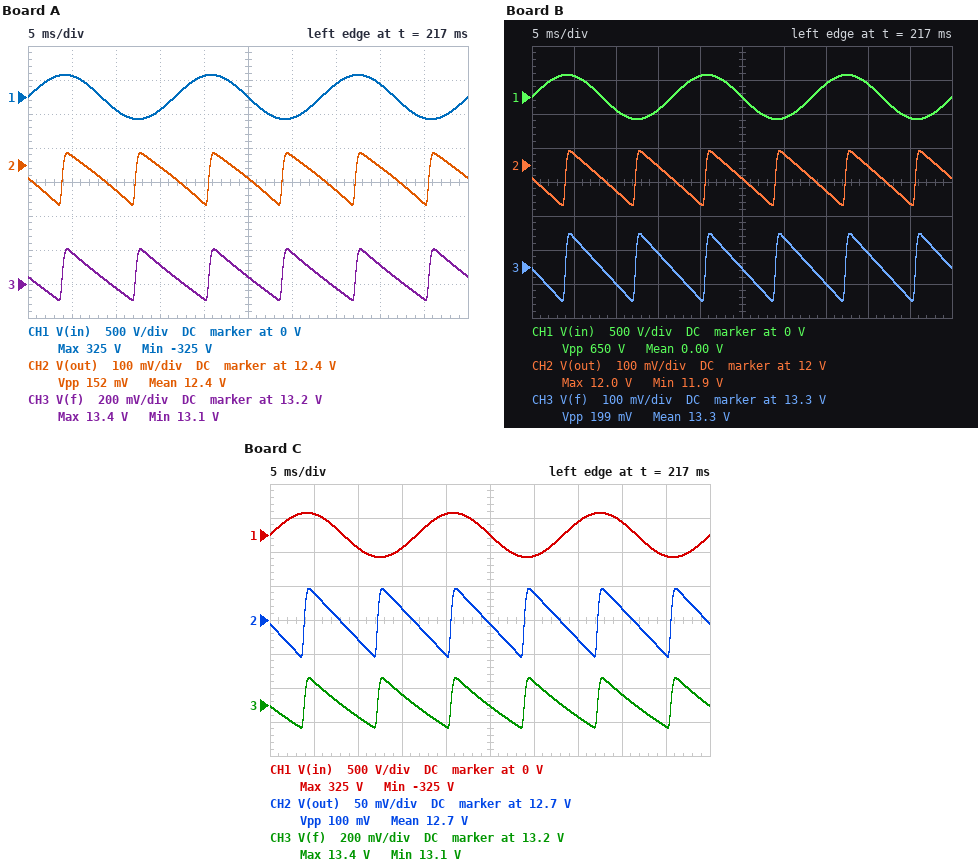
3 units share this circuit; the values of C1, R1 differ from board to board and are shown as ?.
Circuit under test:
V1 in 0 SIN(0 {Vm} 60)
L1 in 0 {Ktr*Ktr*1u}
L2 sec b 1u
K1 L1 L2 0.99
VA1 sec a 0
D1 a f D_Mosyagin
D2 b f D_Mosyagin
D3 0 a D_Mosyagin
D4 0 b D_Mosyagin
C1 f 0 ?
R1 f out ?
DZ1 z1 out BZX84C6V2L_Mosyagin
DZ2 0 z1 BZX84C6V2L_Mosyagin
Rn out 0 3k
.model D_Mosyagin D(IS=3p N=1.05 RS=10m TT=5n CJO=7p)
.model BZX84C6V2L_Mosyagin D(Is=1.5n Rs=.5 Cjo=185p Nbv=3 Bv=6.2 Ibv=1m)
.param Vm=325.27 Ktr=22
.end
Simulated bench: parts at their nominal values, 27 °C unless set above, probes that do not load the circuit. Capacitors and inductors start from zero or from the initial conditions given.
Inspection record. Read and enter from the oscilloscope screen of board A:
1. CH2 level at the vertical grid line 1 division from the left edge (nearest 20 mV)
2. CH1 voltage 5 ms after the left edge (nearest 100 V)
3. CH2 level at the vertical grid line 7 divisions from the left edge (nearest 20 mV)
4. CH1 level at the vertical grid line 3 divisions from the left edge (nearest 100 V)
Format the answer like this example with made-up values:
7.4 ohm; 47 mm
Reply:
12.42 V; 300 V; 12.32 V; -200 V
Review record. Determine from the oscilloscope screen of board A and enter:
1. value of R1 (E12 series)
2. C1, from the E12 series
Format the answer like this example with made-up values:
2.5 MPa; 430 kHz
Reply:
180 Ω; 120 µF
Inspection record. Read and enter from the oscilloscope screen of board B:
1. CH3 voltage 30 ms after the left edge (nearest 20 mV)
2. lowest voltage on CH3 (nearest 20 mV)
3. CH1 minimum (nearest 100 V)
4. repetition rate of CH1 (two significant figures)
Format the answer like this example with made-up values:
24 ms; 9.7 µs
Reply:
13.38 V; 13.20 V; -300 V; 60 Hz
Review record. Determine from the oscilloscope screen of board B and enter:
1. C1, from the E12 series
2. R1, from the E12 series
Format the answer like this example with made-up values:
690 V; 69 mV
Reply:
150 µF; 330 Ω
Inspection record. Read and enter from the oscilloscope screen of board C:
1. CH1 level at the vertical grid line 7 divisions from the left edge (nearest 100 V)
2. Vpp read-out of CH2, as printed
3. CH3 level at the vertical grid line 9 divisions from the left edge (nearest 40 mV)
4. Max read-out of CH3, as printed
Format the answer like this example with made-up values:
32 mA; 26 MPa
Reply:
200 V; 100 mV; 13.08 V; 13.4 V
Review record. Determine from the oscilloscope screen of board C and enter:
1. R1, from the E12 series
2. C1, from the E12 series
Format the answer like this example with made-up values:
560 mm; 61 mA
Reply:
47 Ω; 270 µF
